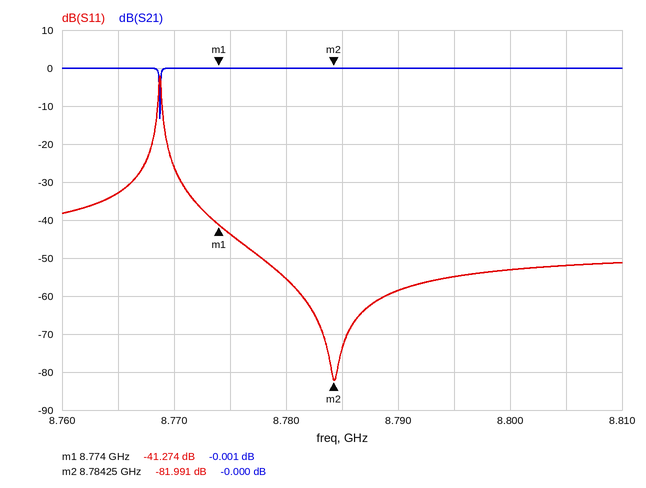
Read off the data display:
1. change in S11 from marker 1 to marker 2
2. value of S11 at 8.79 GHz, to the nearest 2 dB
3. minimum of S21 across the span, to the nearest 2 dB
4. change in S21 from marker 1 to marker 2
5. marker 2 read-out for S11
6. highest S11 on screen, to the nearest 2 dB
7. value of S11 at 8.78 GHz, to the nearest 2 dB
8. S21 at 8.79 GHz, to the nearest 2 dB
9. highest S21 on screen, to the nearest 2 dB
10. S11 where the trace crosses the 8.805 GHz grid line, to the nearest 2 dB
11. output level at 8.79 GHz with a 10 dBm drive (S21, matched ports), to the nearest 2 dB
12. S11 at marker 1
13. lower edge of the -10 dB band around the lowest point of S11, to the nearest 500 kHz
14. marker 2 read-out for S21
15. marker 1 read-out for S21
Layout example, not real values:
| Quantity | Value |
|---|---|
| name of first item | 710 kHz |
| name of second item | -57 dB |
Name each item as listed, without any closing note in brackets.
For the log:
| Quantity | Value |
|---|---|
| change in S11 from marker 1 to marker 2 | -40.717 dB |
| value of S11 at 8.79 GHz, to the nearest 2 dB | -58 dB |
| minimum of S21 across the span, to the nearest 2 dB | -14 dB |
| change in S21 from marker 1 to marker 2 | 0.001 dB |
| marker 2 read-out for S11 | -81.991 dB |
| highest S11 on screen, to the nearest 2 dB | -2 dB |
| value of S11 at 8.78 GHz, to the nearest 2 dB | -56 dB |
| S21 at 8.79 GHz, to the nearest 2 dB | 0 dB |
| highest S21 on screen, to the nearest 2 dB | 0 dB |
| S11 where the trace crosses the 8.805 GHz grid line, to the nearest 2 dB | -52 dB |
| output level at 8.79 GHz with a 10 dBm drive (S21, matched ports), to the nearest 2 dB | 10 dBm |
| S11 at marker 1 | -41.274 dB |
| lower edge of the -10 dB band around the lowest point of S11, to the nearest 500 kHz | 8.7690 GHz |
| marker 2 read-out for S21 | -0.000 dB |
| marker 1 read-out for S21 | -0.001 dB |
